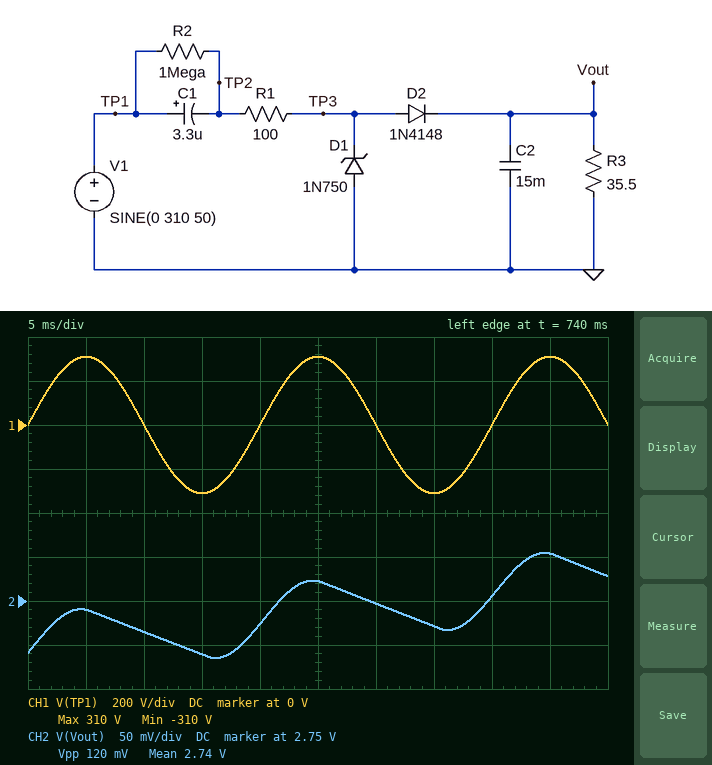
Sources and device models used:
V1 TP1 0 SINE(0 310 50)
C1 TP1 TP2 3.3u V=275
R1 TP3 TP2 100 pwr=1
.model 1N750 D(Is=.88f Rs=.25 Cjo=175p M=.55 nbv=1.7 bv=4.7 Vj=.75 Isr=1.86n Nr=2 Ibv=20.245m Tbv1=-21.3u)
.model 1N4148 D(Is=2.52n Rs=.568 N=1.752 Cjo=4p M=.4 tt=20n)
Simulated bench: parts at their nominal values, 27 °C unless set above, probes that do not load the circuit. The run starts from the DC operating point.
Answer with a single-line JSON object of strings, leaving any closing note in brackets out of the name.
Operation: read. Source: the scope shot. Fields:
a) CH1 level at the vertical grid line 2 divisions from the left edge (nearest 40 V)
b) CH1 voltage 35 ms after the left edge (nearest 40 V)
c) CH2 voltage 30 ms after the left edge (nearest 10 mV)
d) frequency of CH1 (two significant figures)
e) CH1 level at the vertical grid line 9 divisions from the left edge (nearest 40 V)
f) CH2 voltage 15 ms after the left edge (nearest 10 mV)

{"CH1 level at the vertical grid line 2 divisions from the left edge": "0 V", "CH1 voltage 35 ms after the left edge": "-320 V", "CH2 voltage 30 ms after the left edge": "2.75 V", "frequency of CH1": "50 Hz", "CH1 level at the vertical grid line 9 divisions from the left edge": "320 V", "CH2 voltage 15 ms after the left edge": "2.69 V"}
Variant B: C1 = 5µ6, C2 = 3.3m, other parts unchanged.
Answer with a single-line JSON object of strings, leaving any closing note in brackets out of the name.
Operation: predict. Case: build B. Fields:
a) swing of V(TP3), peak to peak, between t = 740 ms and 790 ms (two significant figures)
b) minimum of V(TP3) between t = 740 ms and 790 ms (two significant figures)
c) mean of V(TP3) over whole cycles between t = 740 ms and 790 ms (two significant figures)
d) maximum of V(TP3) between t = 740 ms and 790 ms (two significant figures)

{"swing of V(TP3), peak to peak, between t = 740 ms and 790 ms": "5.9 V", "minimum of V(TP3) between t = 740 ms and 790 ms": "-1.0 V", "mean of V(TP3) over whole cycles between t = 740 ms and 790 ms": "1.9 V", "maximum of V(TP3) between t = 740 ms and 790 ms": "4.9 V"}
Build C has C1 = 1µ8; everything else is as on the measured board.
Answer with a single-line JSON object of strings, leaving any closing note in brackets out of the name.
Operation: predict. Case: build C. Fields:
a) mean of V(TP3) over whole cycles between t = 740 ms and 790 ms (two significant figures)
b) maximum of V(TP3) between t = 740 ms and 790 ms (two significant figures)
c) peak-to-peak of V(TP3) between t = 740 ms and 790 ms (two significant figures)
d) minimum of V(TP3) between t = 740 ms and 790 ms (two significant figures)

{"mean of V(TP3) over whole cycles between t = 740 ms and 790 ms": "740 mV", "maximum of V(TP3) between t = 740 ms and 790 ms": "2.4 V", "peak-to-peak of V(TP3) between t = 740 ms and 790 ms": "3.3 V", "minimum of V(TP3) between t = 740 ms and 790 ms": "-890 mV"}
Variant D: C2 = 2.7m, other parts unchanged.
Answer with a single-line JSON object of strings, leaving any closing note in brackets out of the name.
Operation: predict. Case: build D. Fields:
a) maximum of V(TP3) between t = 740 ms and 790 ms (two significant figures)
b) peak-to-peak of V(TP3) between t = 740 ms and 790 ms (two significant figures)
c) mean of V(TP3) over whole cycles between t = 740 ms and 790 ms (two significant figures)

{"maximum of V(TP3) between t = 740 ms and 790 ms": "4.7 V", "peak-to-peak of V(TP3) between t = 740 ms and 790 ms": "5.6 V", "mean of V(TP3) over whole cycles between t = 740 ms and 790 ms": "1.8 V"}
